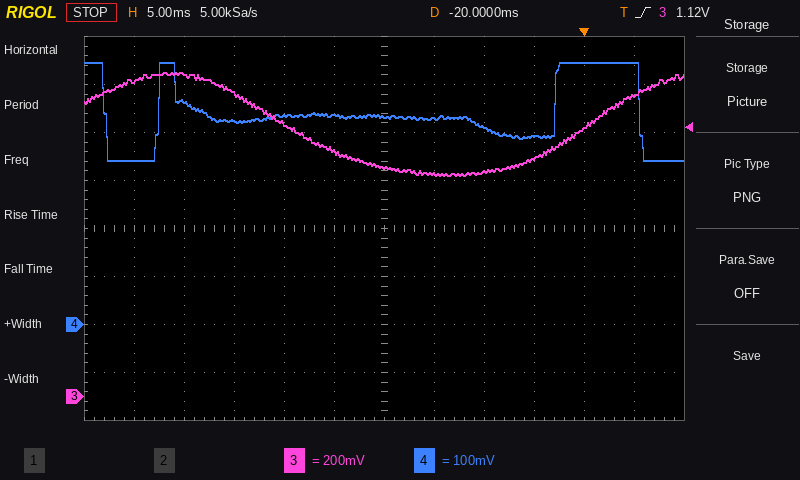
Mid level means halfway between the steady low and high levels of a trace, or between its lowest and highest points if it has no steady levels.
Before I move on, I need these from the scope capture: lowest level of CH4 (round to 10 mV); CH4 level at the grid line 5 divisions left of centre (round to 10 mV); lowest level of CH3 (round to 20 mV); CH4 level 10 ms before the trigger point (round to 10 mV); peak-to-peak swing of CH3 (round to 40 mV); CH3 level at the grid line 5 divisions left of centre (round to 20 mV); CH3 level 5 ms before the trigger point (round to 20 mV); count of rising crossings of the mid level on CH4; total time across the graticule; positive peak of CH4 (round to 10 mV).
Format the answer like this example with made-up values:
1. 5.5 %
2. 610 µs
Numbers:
1. 340 mV
2. 340 mV
3. 920 mV
4. 410 mV
5. 440 mV
6. 1.32 V
7. 1.00 V
8. 2
9. 60 ms
10. 550 mV
